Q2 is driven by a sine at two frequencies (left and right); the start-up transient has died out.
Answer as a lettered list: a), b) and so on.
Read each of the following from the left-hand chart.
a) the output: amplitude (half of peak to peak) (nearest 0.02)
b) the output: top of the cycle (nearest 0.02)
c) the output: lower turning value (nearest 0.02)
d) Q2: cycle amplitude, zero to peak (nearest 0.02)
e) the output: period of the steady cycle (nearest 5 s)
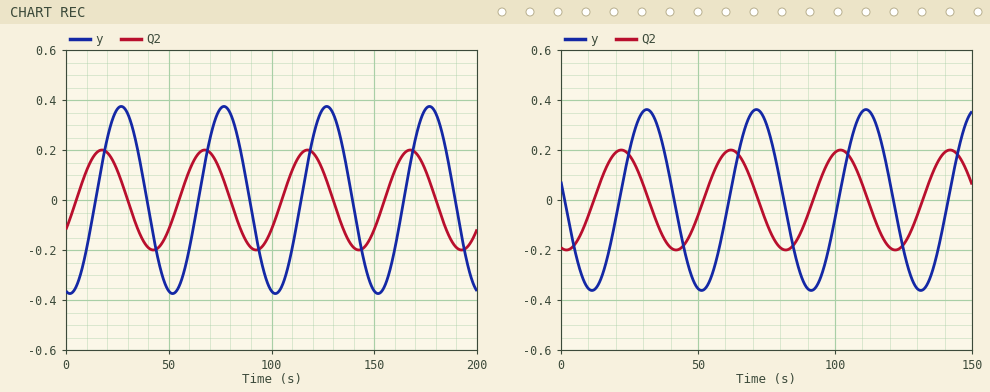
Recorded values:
a) 0.38
b) 0.38
c) -0.38
d) 0.20
e) 50 s
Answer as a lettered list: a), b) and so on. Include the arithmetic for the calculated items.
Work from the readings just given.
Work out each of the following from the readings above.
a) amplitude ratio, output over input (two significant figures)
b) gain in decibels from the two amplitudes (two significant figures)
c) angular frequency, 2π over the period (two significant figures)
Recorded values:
a) 0.38 / 0.2 = 1.9
b) 20 log10(0.38 / 0.2) = 5.6 dB
c) 2π / 50 = 0.13 rad/s
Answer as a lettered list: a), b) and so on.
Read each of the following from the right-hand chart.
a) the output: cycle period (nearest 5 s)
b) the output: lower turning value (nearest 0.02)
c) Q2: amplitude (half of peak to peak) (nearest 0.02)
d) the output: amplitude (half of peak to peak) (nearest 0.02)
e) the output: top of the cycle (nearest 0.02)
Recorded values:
a) 40 s
b) -0.36
c) 0.20
d) 0.36
e) 0.36
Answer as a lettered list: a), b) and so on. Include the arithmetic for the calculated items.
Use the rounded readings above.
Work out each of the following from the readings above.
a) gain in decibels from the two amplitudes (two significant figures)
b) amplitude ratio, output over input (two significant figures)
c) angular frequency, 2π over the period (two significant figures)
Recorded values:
a) 20 log10(0.36 / 0.2) = 5.1 dB
b) 0.36 / 0.2 = 1.8
c) 2π / 40 = 0.16 rad/s
